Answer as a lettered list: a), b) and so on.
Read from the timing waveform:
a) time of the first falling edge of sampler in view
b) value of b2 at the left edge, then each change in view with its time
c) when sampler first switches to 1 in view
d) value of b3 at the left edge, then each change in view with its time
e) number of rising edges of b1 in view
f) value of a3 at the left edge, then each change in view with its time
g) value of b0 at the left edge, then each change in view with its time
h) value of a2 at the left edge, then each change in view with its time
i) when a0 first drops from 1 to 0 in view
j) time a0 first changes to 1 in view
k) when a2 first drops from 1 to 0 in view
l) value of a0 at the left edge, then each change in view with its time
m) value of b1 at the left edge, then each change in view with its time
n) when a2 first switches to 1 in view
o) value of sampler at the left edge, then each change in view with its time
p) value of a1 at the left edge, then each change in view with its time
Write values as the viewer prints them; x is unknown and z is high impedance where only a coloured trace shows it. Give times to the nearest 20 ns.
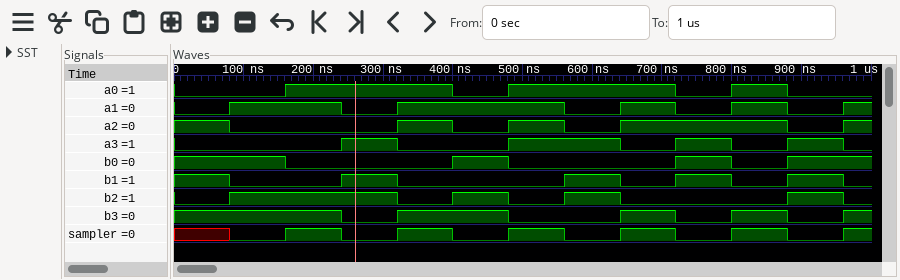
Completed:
a) 240 ns
b) 0, 1 at 80 ns, 0 at 320 ns, 1 at 400 ns, 0 at 480 ns, 1 at 560 ns, 0 at 640 ns, 1 at 880 ns, 0 at 960 ns
c) 160 ns
d) 1, 0 at 240 ns, 1 at 320 ns, 0 at 480 ns, 1 at 640 ns, 0 at 720 ns, 1 at 800 ns, 0 at 880 ns, 1 at 960 ns
e) 4
f) 0, 1 at 240 ns, 0 at 320 ns, 1 at 480 ns, 0 at 640 ns, 1 at 720 ns, 0 at 800 ns, 1 at 880 ns, 0 at 960 ns
g) 1, 0 at 160 ns, 1 at 400 ns, 0 at 480 ns, 1 at 720 ns, 0 at 800 ns, 1 at 880 ns
h) 1, 0 at 80 ns, 1 at 320 ns, 0 at 400 ns, 1 at 480 ns, 0 at 560 ns, 1 at 640 ns, 0 at 880 ns, 1 at 960 ns
i) 400 ns
j) 160 ns
k) 80 ns
l) 0, 1 at 160 ns, 0 at 400 ns, 1 at 480 ns, 0 at 720 ns, 1 at 800 ns, 0 at 880 ns
m) 1, 0 at 80 ns, 1 at 240 ns, 0 at 320 ns, 1 at 560 ns, 0 at 640 ns, 1 at 720 ns, 0 at 800 ns, 1 at 880 ns, 0 at 960 ns
n) 320 ns
o) x, 0 at 80 ns, 1 at 160 ns, 0 at 240 ns, 1 at 320 ns, 0 at 400 ns, 1 at 480 ns, 0 at 560 ns, 1 at 640 ns, 0 at 720 ns, 1 at 800 ns, 0 at 880 ns, 1 at 960 ns
p) 0, 1 at 80 ns, 0 at 240 ns, 1 at 320 ns, 0 at 560 ns, 1 at 640 ns, 0 at 720 ns, 1 at 800 ns, 0 at 880 ns, 1 at 960 ns
